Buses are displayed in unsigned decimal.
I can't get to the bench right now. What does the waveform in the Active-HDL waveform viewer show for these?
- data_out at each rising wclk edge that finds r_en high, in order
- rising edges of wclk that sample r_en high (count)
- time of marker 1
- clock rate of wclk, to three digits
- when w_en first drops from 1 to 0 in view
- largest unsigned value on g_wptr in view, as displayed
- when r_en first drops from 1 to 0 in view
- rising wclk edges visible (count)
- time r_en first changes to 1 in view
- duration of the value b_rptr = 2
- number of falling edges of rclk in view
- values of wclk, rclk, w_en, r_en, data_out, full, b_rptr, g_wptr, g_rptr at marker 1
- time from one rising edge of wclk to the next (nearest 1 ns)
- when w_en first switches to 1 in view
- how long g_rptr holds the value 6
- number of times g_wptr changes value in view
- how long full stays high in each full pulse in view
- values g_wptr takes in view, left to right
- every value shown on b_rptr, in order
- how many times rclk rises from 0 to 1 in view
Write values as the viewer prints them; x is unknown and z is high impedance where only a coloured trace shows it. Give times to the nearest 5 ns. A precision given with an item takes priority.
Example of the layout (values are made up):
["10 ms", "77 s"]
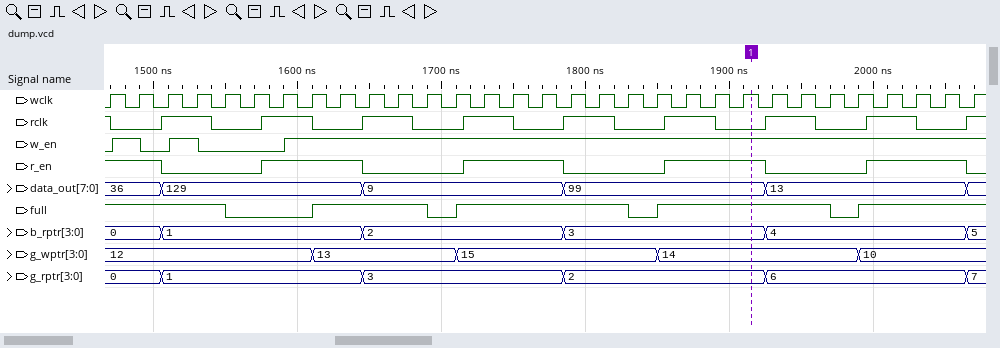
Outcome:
["36, 36, 129, 129, 129, 9, 9, 9, 99, 99, 99, 13, 13, 13", "14", "1915 ns", "50.0 MHz", "1490 ns", "15", "1505 ns", "31", "1575 ns", "140 ns", "9", "wclk=1, rclk=0, w_en=1, r_en=1, data_out=99, full=1, b_rptr=3, g_wptr=14, g_rptr=2", "20 ns", "1470 ns", "140 ns", "4", "80 ns, 120 ns, 120 ns", "12, 13, 15, 14, 10", "0, 1, 2, 3, 4, 5", "9"]
